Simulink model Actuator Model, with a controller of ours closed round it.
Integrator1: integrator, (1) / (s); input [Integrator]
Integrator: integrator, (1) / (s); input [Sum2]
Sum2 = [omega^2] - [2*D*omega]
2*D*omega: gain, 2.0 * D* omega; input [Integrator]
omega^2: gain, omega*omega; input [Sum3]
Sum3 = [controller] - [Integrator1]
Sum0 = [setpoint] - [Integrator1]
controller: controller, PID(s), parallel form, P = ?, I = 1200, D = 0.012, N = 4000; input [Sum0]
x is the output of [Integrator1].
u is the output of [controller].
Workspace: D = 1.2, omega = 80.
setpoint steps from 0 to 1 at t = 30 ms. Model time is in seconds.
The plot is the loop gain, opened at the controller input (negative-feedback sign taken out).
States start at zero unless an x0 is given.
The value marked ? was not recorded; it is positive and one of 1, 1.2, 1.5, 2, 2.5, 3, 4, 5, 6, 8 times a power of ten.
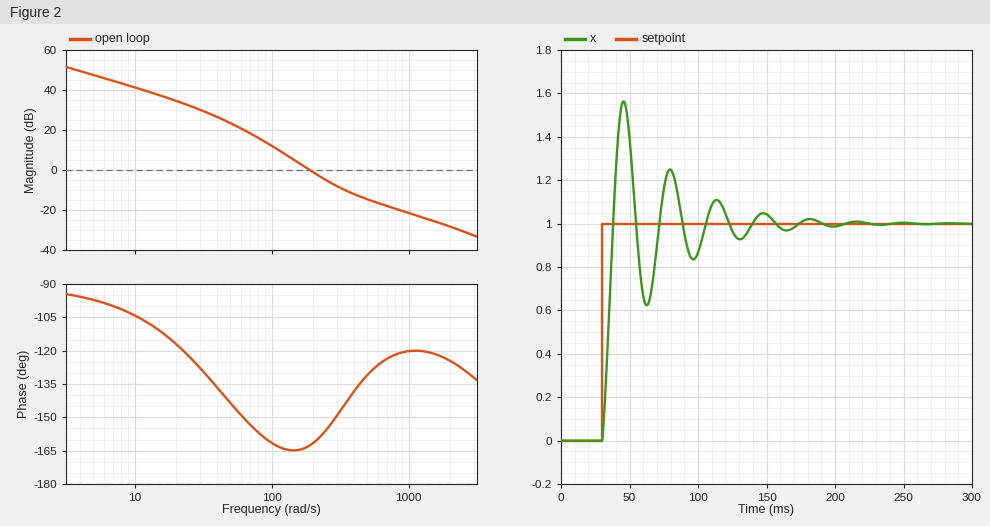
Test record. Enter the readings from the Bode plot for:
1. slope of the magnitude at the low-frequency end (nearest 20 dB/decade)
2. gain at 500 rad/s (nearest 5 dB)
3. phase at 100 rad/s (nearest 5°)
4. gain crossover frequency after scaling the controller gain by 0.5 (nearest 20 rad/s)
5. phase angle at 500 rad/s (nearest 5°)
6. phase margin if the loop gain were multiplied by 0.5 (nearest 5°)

-20 dB/decade
-15 dB
-160°
140 rad/s
-130°
15°
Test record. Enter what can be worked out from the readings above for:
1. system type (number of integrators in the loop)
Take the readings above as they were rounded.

1
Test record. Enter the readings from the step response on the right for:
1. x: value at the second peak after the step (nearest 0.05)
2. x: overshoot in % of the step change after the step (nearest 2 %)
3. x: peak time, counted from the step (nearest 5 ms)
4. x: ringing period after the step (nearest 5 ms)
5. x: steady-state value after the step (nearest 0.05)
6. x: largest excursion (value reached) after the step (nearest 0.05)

1.25
56 %
15 ms
35 ms
1.00
1.55
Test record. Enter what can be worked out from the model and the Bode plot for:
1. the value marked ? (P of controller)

6
